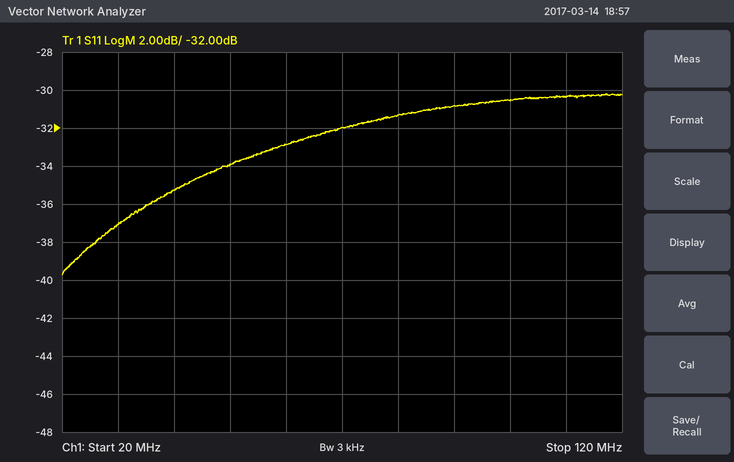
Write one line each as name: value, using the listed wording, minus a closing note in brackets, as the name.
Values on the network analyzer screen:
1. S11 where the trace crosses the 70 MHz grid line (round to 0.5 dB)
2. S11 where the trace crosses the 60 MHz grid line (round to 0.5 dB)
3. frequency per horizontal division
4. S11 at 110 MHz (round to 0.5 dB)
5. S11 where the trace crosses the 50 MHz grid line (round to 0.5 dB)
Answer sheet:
S11 where the trace crosses the 70 MHz grid line: -32.0 dB
S11 where the trace crosses the 60 MHz grid line: -33.0 dB
frequency per horizontal division: 10 MHz
S11 at 110 MHz: -30.5 dB
S11 where the trace crosses the 50 MHz grid line: -34.0 dB
